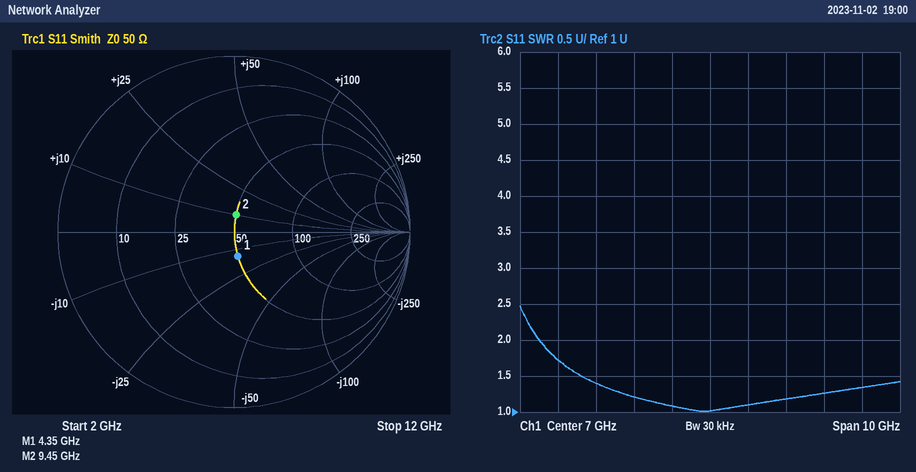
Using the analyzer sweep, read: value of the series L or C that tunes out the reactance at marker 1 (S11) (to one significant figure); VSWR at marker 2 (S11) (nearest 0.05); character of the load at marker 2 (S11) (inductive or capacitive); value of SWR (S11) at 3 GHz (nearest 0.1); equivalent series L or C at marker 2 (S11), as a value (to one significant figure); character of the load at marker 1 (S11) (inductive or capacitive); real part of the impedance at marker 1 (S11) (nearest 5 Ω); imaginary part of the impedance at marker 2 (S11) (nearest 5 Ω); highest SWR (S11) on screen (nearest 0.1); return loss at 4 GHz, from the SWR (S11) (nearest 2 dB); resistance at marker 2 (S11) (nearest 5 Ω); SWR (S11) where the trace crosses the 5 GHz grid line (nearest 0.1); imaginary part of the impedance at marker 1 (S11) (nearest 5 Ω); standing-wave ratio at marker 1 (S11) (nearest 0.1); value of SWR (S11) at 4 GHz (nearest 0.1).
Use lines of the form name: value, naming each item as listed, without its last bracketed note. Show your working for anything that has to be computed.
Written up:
value of the series L or C that tunes out the reactance at marker 1 (S11): L = 15 Ω/(2π × 4.35 GHz) ≈ 549 pH, so 500 pH to one significant figure
VSWR at marker 2 (S11): 1.20
character of the load at marker 2 (S11): inductive
value of SWR (S11) at 3 GHz: 1.7
equivalent series L or C at marker 2 (S11), as a value: L = 10 Ω/(2π × 9.45 GHz) ≈ 168 pH, so 200 pH to one significant figure
character of the load at marker 1 (S11): capacitive
real part of the impedance at marker 1 (S11): 50 Ω
imaginary part of the impedance at marker 2 (S11): +10 Ω
highest SWR (S11) on screen: 2.5
return loss at 4 GHz, from the SWR (S11): −20 log10((1.4 − 1)/(1.4 + 1)) ≈ 16 dB
resistance at marker 2 (S11): 50 Ω
SWR (S11) where the trace crosses the 5 GHz grid line: 1.2
imaginary part of the impedance at marker 1 (S11): -15 Ω
standing-wave ratio at marker 1 (S11): 1.3
value of SWR (S11) at 4 GHz: 1.4
